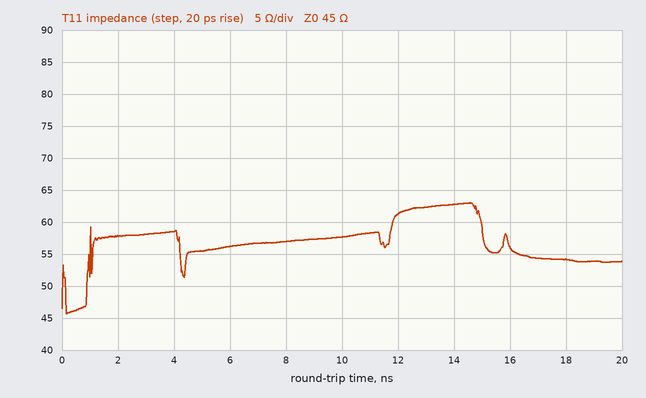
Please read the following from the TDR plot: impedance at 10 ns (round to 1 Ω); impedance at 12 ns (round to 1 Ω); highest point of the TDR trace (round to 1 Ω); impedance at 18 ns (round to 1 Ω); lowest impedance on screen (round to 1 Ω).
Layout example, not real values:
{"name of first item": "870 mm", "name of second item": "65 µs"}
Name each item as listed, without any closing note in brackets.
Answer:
{"impedance at 10 ns": "58 Ω", "impedance at 12 ns": "61 Ω", "highest point of the TDR trace": "63 Ω", "impedance at 18 ns": "54 Ω", "lowest impedance on screen": "46 Ω"}
